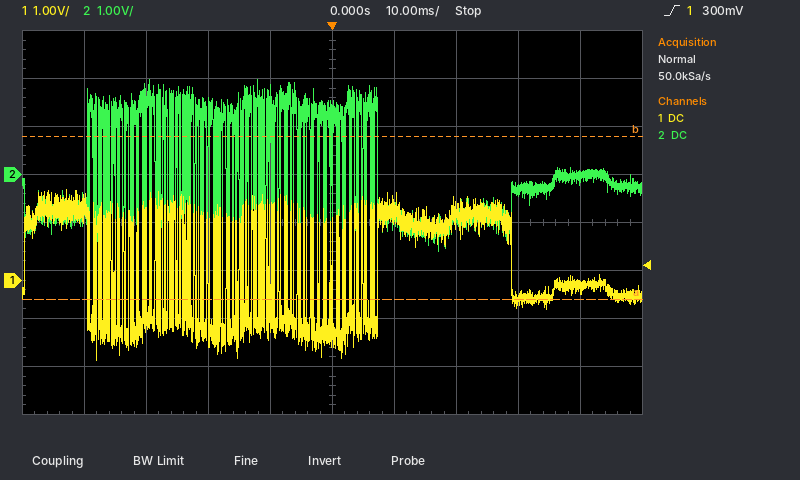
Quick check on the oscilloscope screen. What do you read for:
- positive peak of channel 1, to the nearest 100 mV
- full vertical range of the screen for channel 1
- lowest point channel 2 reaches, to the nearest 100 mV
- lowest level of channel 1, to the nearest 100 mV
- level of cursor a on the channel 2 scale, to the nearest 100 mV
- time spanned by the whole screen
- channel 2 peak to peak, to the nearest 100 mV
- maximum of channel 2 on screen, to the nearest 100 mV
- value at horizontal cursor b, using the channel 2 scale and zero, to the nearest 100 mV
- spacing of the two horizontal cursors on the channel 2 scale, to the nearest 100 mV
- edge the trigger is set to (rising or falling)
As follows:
1.9 V
8 V
-1.6 V
-1.7 V
-2.6 V
100 ms
3.6 V
2.0 V
800 mV
3.4 V
rising
